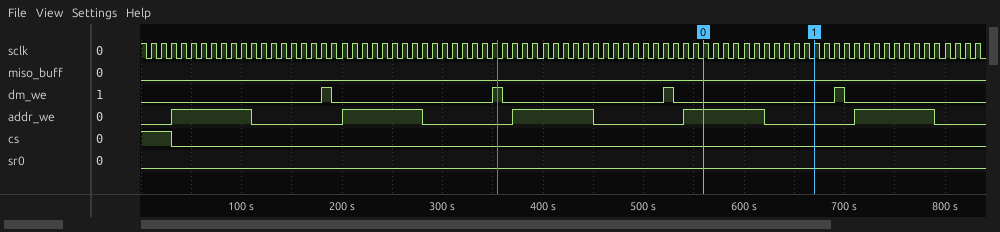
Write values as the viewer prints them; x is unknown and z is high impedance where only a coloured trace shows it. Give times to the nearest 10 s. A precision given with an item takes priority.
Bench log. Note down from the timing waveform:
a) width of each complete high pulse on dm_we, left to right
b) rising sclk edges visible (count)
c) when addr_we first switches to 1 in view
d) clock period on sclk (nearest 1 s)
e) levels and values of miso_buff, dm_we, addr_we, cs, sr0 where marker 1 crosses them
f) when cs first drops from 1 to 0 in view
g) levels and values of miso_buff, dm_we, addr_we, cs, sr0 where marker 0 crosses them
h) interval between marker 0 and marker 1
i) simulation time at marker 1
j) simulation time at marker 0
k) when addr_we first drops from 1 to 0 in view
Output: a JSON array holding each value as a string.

["10 s, 10 s, 10 s, 10 s", "83", "30 s", "10 s", "miso_buff=0, dm_we=0, addr_we=0, cs=0, sr0=0", "30 s", "miso_buff=0, dm_we=0, addr_we=1, cs=0, sr0=0", "110 s", "670 s", "560 s", "110 s"]
